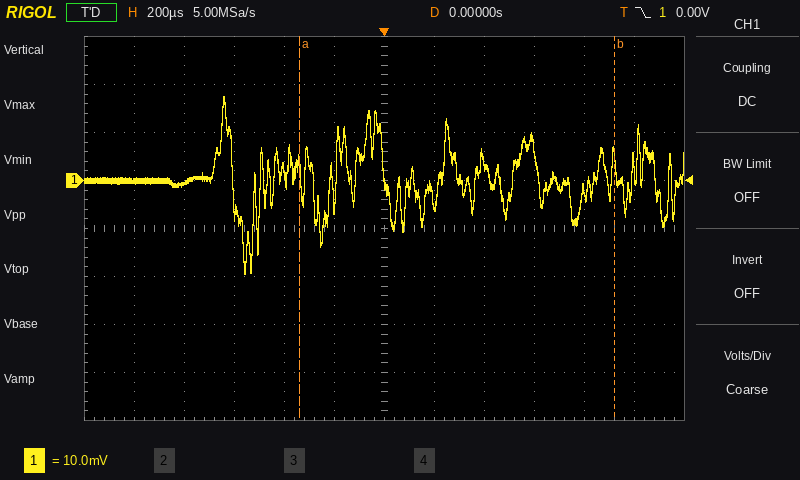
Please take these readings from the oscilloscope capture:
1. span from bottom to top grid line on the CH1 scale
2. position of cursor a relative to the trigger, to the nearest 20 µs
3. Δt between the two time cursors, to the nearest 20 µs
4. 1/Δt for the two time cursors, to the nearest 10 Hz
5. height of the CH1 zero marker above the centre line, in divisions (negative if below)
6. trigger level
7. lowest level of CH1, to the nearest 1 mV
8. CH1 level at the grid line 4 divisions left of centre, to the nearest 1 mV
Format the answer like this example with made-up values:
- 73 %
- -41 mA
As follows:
- 80 mV
- -340 µs
- 1.26 ms
- 790 Hz
- +1.0 div
- 0.00 V
- -19 mV
- -1 mV
